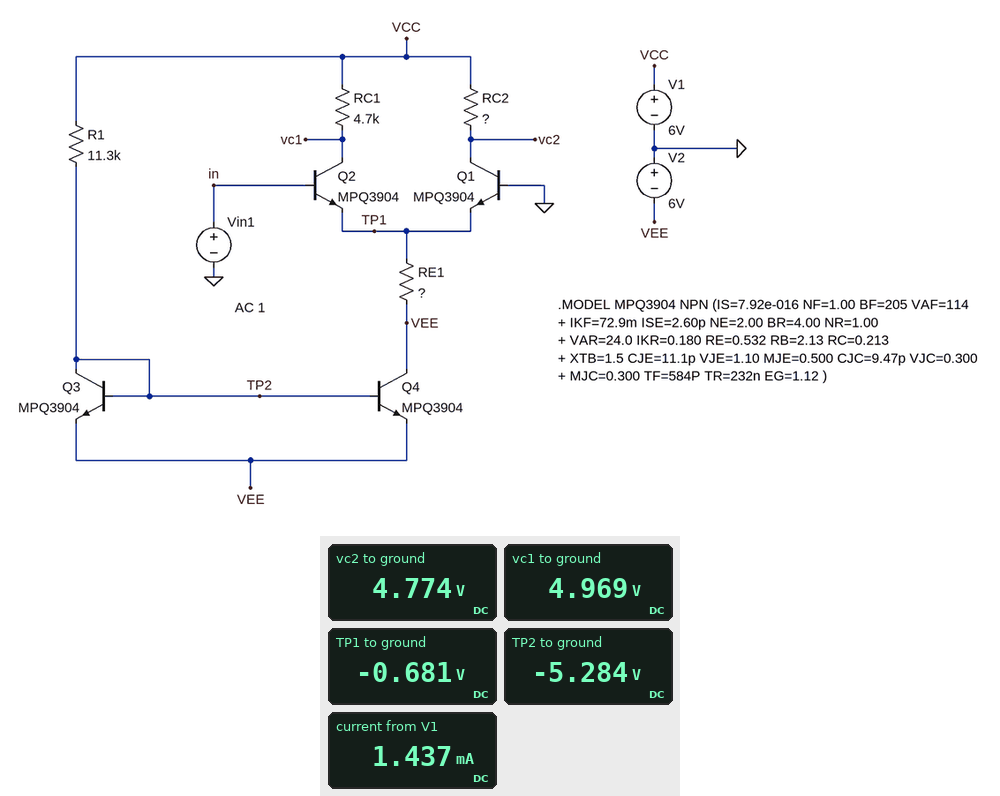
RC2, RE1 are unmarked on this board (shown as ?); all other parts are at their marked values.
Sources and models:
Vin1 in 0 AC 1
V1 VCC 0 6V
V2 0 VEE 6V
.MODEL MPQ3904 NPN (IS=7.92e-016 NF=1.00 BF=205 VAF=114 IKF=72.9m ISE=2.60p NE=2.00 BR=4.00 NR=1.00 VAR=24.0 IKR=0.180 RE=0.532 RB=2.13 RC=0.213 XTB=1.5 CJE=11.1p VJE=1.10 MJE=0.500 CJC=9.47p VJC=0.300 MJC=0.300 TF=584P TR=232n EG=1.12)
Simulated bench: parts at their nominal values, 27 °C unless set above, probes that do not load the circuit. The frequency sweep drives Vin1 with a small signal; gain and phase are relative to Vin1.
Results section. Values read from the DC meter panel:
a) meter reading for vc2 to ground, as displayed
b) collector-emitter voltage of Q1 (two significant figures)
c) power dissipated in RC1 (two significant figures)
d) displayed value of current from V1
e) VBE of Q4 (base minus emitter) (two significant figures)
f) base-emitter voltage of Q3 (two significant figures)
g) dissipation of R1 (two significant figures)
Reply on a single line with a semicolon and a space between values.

4.774 V; 5.5 V; 230 µW; 1.437 mA; 720 mV; 720 mV; 11 mW
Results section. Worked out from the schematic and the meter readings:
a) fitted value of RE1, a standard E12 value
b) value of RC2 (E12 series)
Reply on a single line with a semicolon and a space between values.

12 kΩ; 5.6 kΩ
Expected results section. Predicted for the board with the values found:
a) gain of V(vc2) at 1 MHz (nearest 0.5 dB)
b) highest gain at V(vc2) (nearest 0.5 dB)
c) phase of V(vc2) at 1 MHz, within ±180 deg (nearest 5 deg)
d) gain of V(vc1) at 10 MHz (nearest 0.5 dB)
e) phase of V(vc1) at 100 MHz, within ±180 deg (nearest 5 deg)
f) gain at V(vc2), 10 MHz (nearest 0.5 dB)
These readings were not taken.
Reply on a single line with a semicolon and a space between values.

27.0 dB; 27.5 dB; -10 deg; 22.0 dB; 60 deg; 22.5 dB
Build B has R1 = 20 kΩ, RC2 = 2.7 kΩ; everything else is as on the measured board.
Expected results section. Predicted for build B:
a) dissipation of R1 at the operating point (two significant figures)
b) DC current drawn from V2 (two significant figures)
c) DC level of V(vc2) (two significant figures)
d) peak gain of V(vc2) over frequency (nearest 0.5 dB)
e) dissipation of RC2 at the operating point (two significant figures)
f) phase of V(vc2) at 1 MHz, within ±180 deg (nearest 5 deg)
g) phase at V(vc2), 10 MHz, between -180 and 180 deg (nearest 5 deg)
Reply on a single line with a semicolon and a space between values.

6.4 mW; 1.0 mA; 5.4 V; 21.0 dB; 130 µW; -5 deg; -35 deg
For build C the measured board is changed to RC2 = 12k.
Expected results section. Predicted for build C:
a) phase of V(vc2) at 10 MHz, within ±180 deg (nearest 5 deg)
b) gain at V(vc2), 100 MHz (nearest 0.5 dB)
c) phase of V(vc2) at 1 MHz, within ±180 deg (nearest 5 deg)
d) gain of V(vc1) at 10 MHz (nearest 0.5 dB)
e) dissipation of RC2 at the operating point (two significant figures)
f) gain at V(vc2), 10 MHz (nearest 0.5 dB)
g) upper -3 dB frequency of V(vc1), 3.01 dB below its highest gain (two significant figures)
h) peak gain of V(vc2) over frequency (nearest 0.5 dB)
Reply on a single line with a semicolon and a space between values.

-75 deg; 3.0 dB; -20 deg; 22.0 dB; 570 µW; 23.0 dB; 8.5 MHz; 34.0 dB
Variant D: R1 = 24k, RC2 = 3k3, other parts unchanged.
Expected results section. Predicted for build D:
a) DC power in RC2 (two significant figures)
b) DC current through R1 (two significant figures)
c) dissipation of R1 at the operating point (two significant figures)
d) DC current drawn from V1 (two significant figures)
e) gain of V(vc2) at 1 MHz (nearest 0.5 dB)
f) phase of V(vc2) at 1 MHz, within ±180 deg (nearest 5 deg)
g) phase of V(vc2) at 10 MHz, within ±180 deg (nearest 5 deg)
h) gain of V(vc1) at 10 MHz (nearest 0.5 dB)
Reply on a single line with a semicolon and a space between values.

160 µW; 470 µA; 5.3 mW; 910 µA; 22.5 dB; -5 deg; -40 deg; 22.0 dB
